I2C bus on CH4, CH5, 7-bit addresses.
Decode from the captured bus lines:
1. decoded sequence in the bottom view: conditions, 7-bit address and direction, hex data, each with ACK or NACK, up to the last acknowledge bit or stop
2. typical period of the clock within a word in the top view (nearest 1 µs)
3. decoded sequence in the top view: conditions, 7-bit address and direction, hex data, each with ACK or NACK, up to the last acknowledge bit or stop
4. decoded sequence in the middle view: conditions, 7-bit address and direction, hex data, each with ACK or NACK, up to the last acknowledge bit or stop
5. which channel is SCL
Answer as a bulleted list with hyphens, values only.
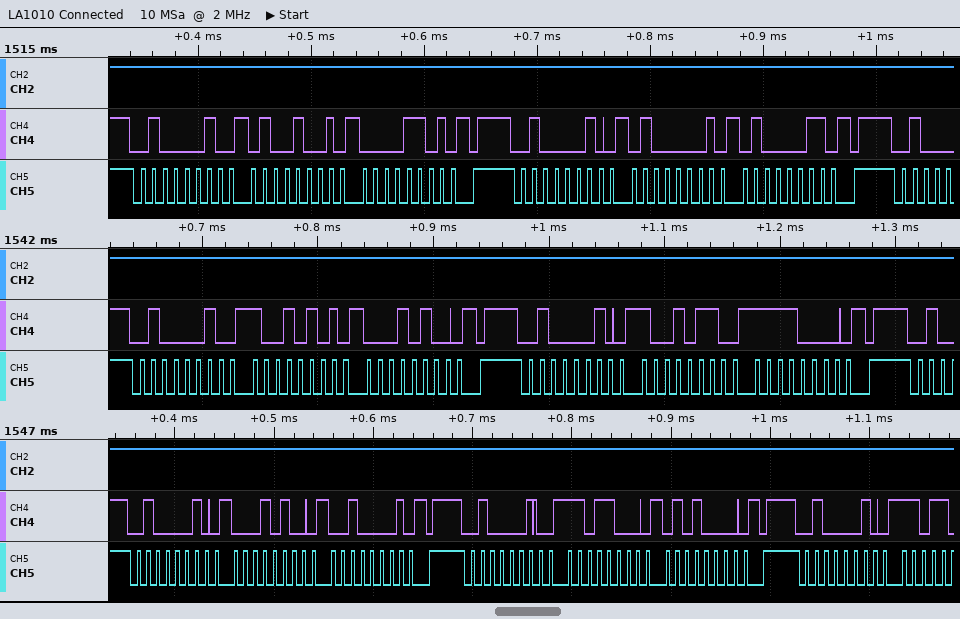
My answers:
- start, address 21 write ACK, 14 ACK, 21 ACK, stop, start, address 21 write ACK, D8 ACK, 50 ACK, stop, start, address 21 write ACK
- 10 µs
- start, address 21 write ACK, 49 ACK, 0D ACK, stop, start, address 21 write ACK, 41 ACK, 43 ACK, stop
- start, address 21 write ACK, 95 ACK, 14 ACK, stop, start, address 21 write ACK, 96 ACK, F0 ACK, stop
- CH5
